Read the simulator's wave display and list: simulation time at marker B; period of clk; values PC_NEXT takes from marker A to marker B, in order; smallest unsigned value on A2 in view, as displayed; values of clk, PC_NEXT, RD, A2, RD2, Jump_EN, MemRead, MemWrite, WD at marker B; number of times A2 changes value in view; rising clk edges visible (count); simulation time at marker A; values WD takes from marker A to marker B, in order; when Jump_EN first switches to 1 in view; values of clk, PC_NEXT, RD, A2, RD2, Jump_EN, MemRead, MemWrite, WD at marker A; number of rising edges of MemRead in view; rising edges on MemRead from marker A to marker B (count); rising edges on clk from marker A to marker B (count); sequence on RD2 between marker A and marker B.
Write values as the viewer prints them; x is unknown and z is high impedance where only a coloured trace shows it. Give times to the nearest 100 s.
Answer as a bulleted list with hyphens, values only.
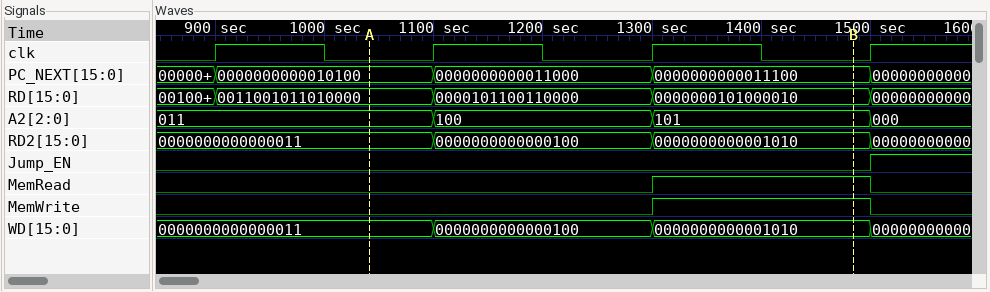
- 1500 s
- 200 s
- 0000000000010100, 0000000000011000, 0000000000011100
- 000
- clk=0, PC_NEXT=0000000000011100, RD=0000000101000010, A2=101, RD2=0000000000001010, Jump_EN=0, MemRead=1, MemWrite=1, WD=0000000000001010
- 3
- 4
- 1000 s
- 0000000000000011, 0000000000000100, 0000000000001010
- 1500 s
- clk=0, PC_NEXT=0000000000010100, RD=0011001011010000, A2=011, RD2=0000000000000011, Jump_EN=0, MemRead=0, MemWrite=0, WD=0000000000000011
- 1
- 1
- 2
- 0000000000000011, 0000000000000100, 0000000000001010
